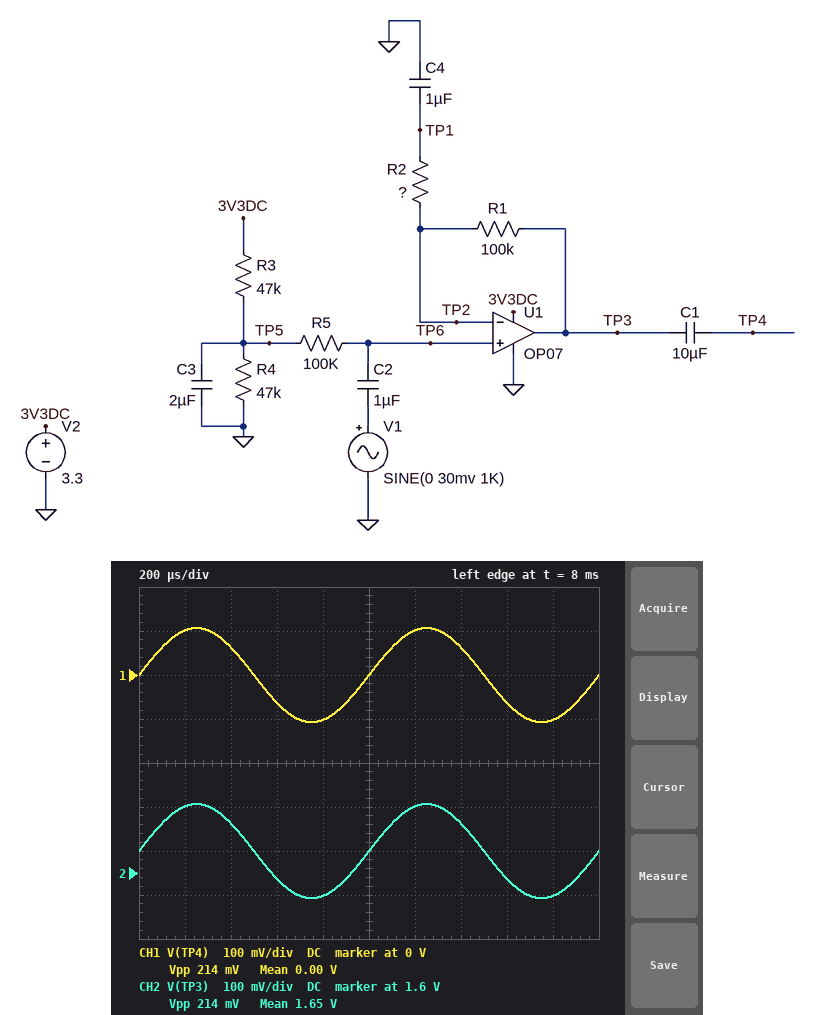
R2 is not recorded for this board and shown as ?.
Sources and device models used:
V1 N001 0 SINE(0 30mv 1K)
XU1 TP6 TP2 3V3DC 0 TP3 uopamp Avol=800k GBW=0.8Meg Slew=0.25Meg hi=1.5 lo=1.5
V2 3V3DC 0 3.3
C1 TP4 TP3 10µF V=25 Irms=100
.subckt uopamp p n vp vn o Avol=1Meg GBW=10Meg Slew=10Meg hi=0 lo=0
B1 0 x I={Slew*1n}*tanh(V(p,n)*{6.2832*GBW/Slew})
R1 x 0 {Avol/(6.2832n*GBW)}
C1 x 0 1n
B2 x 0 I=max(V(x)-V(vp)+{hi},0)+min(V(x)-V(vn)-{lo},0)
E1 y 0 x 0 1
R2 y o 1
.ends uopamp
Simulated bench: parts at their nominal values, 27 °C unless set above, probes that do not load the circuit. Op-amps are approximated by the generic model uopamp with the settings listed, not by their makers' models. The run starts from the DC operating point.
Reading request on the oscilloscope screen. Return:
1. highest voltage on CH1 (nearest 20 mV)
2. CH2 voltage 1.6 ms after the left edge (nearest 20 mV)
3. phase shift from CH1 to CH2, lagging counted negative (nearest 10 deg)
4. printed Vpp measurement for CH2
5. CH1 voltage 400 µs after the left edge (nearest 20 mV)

100 mV
1.58 V
0 deg
214 mV
60 mV
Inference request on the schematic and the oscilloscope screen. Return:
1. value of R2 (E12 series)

39 kΩ
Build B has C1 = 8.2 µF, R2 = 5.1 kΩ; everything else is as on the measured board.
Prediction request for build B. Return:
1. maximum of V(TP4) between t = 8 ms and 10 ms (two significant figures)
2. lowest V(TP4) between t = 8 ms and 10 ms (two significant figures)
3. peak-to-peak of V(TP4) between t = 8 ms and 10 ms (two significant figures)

150 mV
-150 mV
300 mV
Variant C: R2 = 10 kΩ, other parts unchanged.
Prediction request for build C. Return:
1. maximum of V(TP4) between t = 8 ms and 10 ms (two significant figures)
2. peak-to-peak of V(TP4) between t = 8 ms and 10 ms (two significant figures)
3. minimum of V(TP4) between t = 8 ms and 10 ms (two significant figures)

150 mV
300 mV
-150 mV
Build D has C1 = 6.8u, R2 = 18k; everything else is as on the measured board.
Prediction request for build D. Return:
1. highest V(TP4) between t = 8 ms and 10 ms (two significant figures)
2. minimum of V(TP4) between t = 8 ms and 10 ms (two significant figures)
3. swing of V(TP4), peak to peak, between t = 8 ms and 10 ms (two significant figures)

150 mV
-150 mV
300 mV
